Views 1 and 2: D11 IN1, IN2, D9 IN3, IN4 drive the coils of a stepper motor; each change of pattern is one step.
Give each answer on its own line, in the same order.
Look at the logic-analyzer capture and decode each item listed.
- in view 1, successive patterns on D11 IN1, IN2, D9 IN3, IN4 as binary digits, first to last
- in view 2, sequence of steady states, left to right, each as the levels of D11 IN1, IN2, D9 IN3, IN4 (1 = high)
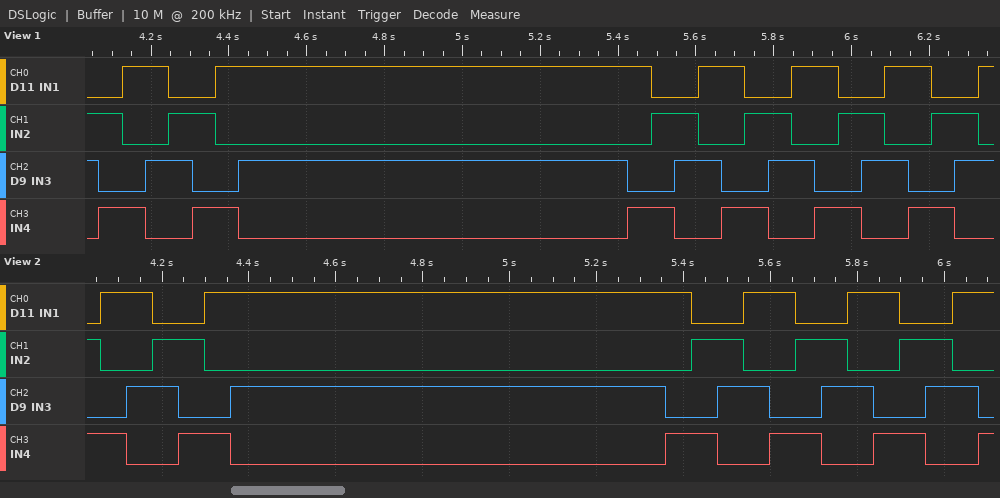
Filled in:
0110 0101 1001 1010 0110 0101 1001 1010 1001 0101 0110 1010 1001 0101 0110 1010 1001 0101 0110 1010 1001 0101 0110 1010
0101 1001 1010 0110 0101 1001 1010 1001 0101 0110 1010 1001 0101 0110 1010 1001 0101 0110 1010 1001
